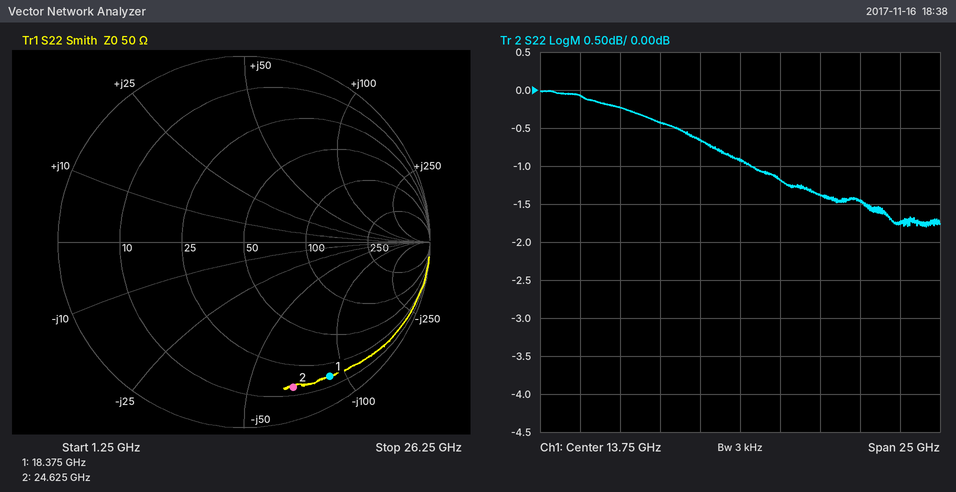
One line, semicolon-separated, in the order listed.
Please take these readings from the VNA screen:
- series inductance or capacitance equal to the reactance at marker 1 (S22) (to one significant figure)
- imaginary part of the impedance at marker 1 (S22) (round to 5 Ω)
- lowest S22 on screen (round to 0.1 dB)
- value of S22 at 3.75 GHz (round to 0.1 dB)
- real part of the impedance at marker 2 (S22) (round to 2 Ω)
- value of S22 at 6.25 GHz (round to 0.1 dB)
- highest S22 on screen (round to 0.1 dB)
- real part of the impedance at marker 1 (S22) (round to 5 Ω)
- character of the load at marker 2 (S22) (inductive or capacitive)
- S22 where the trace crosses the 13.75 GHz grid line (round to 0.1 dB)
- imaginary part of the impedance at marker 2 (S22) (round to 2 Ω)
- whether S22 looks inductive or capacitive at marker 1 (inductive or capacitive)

100 fF; -90 Ω; -1.8 dB; -0.1 dB; 14 Ω; -0.2 dB; 0.0 dB; 15 Ω; capacitive; -0.9 dB; -68 Ω; capacitive
